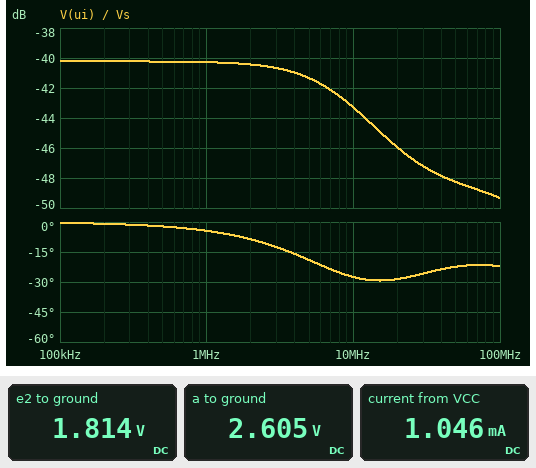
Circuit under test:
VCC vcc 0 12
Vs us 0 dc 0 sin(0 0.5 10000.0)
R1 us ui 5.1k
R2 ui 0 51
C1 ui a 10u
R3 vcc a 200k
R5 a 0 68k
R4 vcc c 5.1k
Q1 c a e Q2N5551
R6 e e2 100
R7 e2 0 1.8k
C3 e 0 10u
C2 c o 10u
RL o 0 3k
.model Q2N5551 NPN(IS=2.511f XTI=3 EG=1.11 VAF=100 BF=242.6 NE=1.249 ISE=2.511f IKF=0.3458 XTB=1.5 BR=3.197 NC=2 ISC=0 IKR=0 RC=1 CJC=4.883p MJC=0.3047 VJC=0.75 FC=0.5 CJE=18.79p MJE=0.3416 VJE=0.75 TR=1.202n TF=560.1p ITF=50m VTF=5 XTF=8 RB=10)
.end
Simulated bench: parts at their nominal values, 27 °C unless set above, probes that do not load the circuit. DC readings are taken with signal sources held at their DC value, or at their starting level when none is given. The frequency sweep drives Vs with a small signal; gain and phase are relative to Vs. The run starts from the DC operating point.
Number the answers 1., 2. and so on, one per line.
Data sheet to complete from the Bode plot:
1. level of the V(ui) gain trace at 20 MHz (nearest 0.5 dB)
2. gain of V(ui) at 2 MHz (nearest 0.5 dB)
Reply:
1. -46.0 dB
2. -40.5 dB
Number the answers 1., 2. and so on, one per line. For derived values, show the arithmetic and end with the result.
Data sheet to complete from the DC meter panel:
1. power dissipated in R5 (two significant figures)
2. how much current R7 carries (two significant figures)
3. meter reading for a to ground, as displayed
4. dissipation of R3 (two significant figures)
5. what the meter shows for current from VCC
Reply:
1. (2.605 V)^2 / 68 kΩ = 100 µW
2. (1.814 V) / 1.8 kΩ = 1.0 mA
3. 2.605 V
4. (12 V - 2.605 V)^2 / 200 kΩ = 440 µW
5. 1.046 mA
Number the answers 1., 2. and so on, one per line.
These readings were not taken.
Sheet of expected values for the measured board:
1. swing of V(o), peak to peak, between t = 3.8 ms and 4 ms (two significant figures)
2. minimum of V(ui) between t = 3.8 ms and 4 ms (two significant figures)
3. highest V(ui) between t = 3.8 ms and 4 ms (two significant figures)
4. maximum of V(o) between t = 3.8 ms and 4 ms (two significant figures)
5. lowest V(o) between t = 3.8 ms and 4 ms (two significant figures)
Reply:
1. 690 mV
2. -4.9 mV
3. 4.9 mV
4. 330 mV
5. -360 mV
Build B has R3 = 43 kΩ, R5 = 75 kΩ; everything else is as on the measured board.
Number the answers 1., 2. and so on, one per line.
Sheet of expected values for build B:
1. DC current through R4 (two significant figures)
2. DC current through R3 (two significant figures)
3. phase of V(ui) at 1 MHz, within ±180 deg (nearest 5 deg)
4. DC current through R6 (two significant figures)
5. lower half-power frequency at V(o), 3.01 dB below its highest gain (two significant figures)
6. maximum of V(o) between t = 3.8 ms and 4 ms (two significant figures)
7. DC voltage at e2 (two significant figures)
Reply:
1. 1.7 mA
2. 180 µA
3. 0 deg
4. 1.8 mA
5. 290 Hz
6. 10 mV
7. 3.2 V
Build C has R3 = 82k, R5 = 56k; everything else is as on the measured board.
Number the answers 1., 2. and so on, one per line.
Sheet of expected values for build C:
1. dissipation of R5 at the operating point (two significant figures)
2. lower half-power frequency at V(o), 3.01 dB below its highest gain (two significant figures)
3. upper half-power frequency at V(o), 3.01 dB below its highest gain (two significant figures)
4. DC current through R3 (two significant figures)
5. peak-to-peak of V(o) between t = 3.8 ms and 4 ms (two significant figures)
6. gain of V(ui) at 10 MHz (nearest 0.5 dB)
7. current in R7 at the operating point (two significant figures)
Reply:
1. 280 µW
2. 370 Hz
3. 13 MHz
4. 98 µA
5. 330 mV
6. -45.5 dB
7. 1.7 mA
